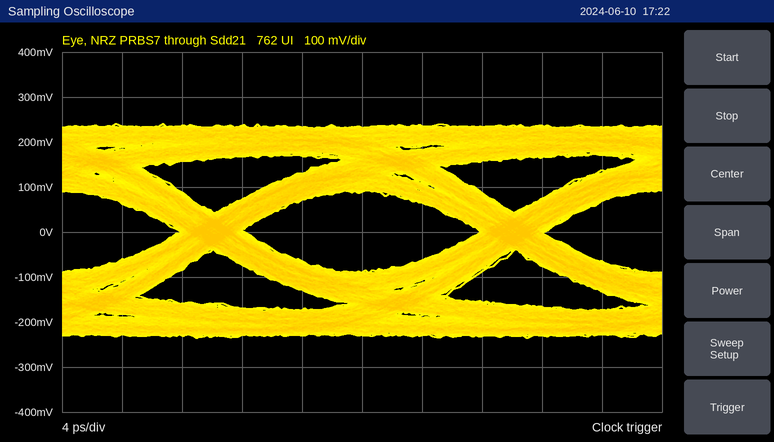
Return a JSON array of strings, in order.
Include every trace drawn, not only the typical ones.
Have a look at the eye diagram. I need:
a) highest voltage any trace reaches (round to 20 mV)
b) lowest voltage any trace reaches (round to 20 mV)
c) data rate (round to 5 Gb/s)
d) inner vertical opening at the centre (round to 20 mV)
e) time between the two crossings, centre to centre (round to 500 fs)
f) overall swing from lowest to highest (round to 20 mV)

["240 mV", "-240 mV", "50 Gb/s", "180 mV", "20.0 ps", "480 mV"]
